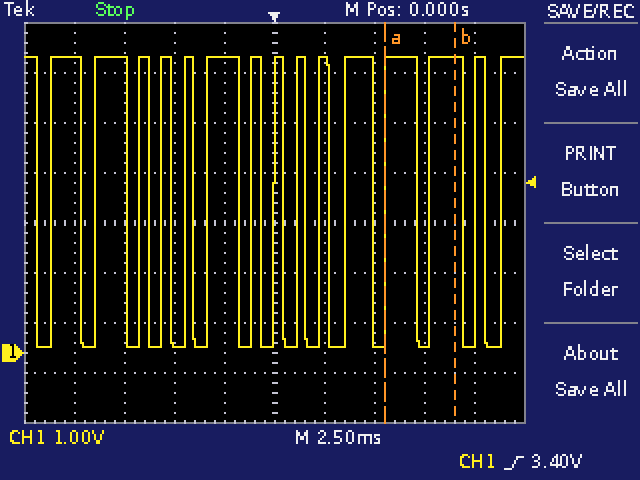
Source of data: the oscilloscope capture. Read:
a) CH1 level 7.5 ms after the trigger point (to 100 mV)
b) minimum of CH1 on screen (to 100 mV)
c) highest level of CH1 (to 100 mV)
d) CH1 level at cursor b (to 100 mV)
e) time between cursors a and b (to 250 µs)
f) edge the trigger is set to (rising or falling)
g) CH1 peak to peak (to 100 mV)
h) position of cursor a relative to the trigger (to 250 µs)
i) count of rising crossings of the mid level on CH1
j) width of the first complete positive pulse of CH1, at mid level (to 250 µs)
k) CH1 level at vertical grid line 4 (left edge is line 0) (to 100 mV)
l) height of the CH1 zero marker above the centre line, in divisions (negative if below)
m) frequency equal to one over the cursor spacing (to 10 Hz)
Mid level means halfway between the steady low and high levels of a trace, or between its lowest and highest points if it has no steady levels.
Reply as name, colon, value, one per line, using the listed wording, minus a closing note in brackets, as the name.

CH1 level 7.5 ms after the trigger point: 100 mV
minimum of CH1 on screen: 100 mV
highest level of CH1: 5.9 V
CH1 level at cursor b: 5.9 V
time between cursors a and b: 3.50 ms
edge the trigger is set to: rising
CH1 peak to peak: 5.8 V
position of cursor a relative to the trigger: +5.50 ms
count of rising crossings of the mid level on CH1: 15
width of the first complete positive pulse of CH1, at mid level: 1.50 ms
CH1 level at vertical grid line 4 (left edge is line 0): 5.9 V
height of the CH1 zero marker above the centre line, in divisions: -2.6 div
frequency equal to one over the cursor spacing: 290 Hz
